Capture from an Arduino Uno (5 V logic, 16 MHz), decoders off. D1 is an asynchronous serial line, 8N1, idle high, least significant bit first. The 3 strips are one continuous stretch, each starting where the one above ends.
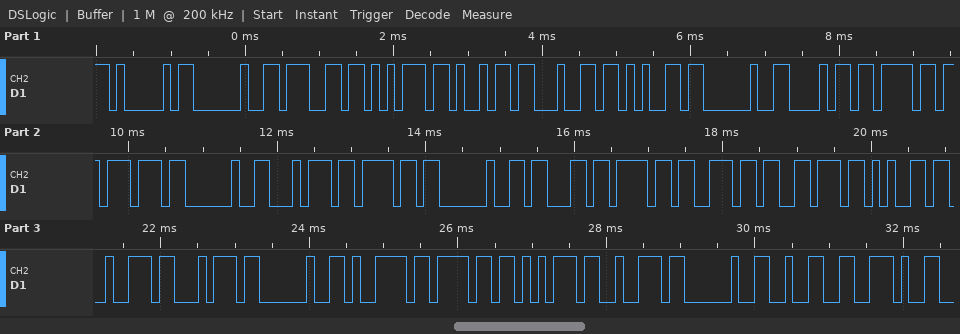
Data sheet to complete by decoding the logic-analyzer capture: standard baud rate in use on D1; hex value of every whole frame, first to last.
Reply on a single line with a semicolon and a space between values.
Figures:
9600 baud; 41 20 67 75 69 64 65 20 68 6F 77 20 74 6F 20 63 6F 6E 76 65 72 74 20 79 6F 75 72 20 32 2E
